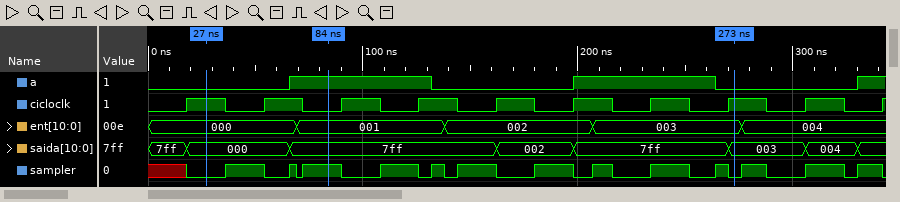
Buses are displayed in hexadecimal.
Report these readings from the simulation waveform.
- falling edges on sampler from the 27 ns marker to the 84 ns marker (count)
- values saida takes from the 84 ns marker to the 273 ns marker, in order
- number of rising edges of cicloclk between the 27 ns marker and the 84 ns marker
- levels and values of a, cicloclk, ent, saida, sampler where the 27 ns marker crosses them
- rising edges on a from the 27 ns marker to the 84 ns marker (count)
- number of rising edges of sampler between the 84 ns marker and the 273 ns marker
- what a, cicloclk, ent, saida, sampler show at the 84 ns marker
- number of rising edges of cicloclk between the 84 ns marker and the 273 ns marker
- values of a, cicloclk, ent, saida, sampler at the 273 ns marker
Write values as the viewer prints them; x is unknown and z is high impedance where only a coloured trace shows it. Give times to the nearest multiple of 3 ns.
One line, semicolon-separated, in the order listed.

2; 7ff, 002, 7ff, 003; 1; a=0, cicloclk=1, ent=000, saida=000, sampler=0; 1; 7; a=1, cicloclk=0, ent=001, saida=7ff, sampler=1; 6; a=0, cicloclk=1, ent=003, saida=003, sampler=0
